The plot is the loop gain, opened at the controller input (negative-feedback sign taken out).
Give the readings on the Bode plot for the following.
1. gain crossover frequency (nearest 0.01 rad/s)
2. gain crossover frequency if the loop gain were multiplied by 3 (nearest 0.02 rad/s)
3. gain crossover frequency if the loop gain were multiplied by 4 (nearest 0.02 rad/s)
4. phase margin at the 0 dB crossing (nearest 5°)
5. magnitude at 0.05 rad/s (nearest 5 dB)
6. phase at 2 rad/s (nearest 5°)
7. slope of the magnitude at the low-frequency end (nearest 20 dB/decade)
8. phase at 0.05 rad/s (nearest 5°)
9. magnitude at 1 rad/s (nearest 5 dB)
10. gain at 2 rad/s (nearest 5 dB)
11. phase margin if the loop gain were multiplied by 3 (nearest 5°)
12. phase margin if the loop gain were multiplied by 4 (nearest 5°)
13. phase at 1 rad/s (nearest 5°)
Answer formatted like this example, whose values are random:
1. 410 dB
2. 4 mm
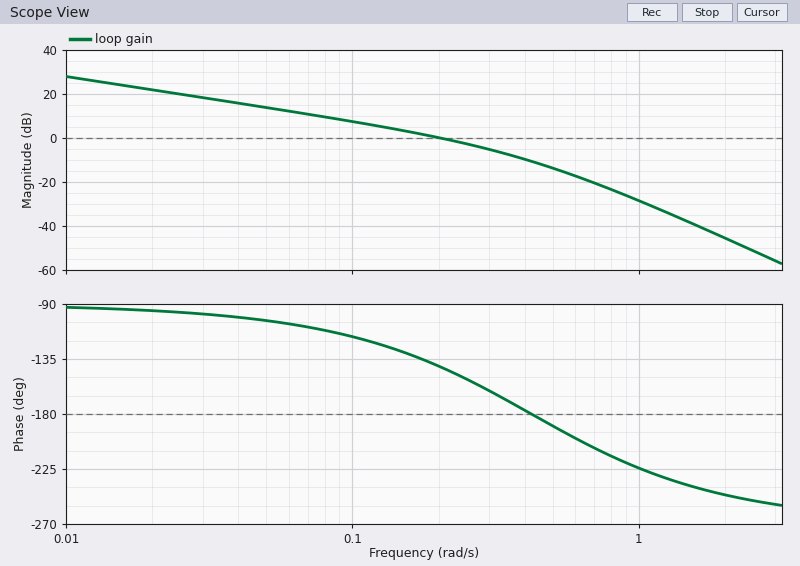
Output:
1. 0.20 rad/s
2. 0.40 rad/s
3. 0.46 rad/s
4. 40°
5. 15 dB
6. -245°
7. -20 dB/decade
8. -105°
9. -30 dB
10. -45 dB
11. 5°
12. -5°
13. -225°
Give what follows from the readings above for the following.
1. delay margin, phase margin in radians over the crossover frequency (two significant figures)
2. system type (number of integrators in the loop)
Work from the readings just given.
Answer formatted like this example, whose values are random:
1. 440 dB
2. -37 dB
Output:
1. 3.5 s
2. 1
